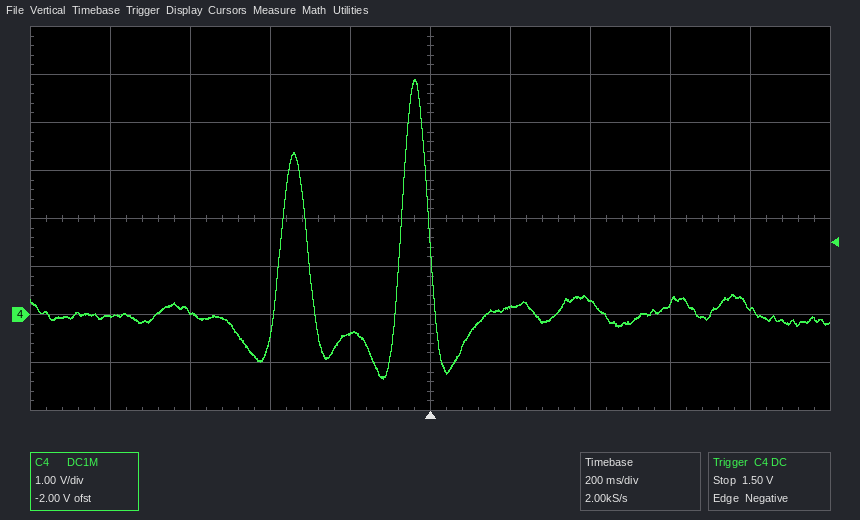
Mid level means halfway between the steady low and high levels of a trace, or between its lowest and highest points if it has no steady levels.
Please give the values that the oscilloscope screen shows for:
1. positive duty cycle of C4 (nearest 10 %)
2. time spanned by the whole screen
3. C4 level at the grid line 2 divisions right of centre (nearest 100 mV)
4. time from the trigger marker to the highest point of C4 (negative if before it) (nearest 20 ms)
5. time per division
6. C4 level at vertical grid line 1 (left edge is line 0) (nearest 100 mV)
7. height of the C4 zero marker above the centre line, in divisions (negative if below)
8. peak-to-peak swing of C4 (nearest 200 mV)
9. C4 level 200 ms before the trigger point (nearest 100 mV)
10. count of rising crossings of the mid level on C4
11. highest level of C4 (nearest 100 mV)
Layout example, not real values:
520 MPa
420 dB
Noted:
20 %
2 s
300 mV
-40 ms
200 ms
0.0 V
-2.0 div
6.2 V
-400 mV
2
4.9 V
